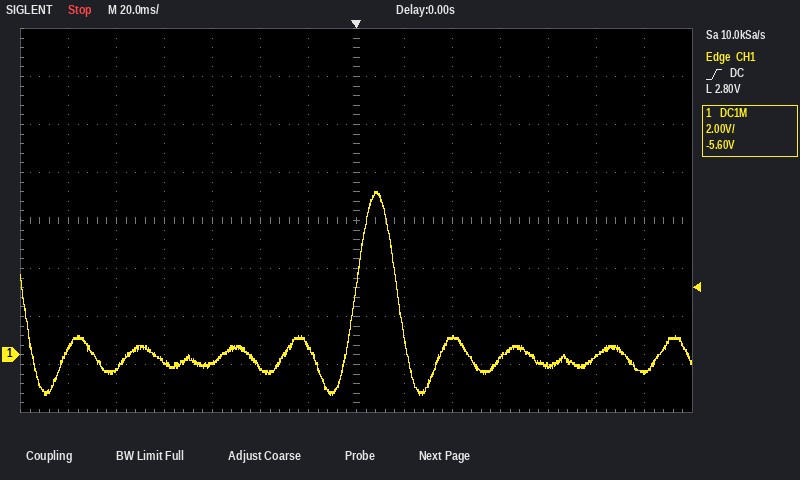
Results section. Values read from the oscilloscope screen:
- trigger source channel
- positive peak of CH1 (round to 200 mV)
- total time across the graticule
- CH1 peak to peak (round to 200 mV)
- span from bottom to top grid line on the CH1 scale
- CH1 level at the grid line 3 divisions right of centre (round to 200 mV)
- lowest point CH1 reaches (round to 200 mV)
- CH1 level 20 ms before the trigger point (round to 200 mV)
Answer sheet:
CH1
6.8 V
280 ms
8.4 V
16 V
-200 mV
-1.6 V
400 mV
